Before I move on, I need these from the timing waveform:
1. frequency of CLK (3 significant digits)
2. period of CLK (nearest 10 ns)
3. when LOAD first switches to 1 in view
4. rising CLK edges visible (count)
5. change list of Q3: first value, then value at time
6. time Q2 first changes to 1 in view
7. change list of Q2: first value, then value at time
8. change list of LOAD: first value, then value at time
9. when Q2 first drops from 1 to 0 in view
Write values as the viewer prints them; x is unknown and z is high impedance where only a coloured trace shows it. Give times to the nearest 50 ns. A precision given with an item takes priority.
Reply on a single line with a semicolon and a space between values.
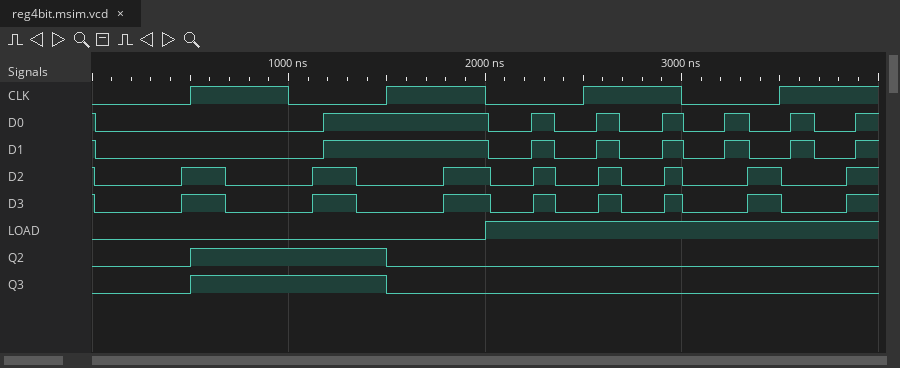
1.00 MHz; 1000 ns; 2000 ns; 4; 0, 1 at 500 ns, 0 at 1500 ns; 500 ns; 0, 1 at 500 ns, 0 at 1500 ns; 0, 1 at 2000 ns; 1500 ns
